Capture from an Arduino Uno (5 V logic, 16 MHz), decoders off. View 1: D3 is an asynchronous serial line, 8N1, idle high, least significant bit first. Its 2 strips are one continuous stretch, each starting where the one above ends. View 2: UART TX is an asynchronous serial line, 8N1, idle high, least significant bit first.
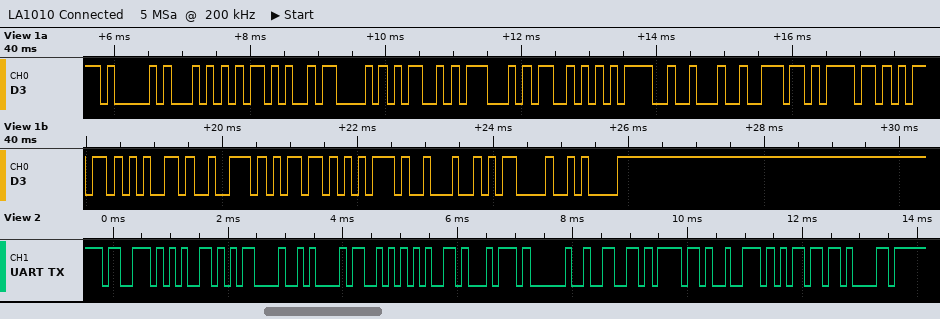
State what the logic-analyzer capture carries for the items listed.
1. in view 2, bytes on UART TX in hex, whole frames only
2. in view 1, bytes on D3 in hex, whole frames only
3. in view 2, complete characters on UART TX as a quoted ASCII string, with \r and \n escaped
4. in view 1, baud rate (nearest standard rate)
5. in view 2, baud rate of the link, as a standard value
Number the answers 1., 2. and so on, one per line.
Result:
1. 73 65 0D 0A 53 65 74 20 66 6F 72 6D 61
2. 41 54 2B 43 4D 47 53 3D 22 6E 6F 6D 65 72 6D 75 22 0D 0A
3. "se\r\nSet forma"
4. 9600 baud
5. 9600 baud
